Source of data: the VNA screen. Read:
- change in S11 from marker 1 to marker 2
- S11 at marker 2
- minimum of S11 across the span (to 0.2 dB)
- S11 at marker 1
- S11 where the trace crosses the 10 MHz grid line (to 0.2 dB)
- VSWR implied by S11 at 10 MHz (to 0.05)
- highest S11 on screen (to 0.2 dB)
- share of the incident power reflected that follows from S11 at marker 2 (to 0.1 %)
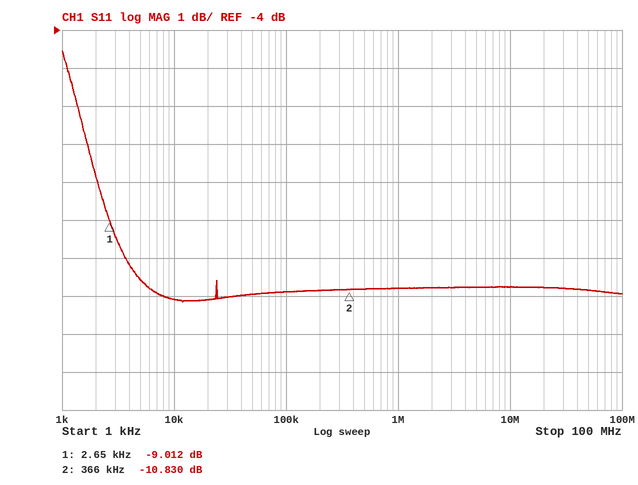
-1.818 dB
-10.830 dB
-11.2 dB
-9.012 dB
-10.8 dB
1.80
-4.6 dB
8.3 %
